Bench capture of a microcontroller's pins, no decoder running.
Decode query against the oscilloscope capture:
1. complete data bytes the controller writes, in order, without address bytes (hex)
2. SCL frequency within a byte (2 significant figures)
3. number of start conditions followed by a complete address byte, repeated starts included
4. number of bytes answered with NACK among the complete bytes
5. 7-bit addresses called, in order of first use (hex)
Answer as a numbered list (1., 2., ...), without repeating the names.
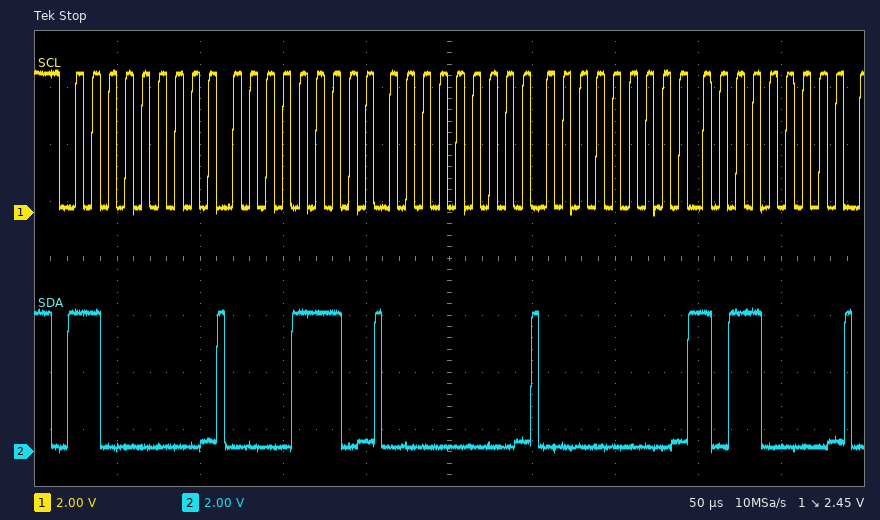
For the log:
1. 0E 00 00 B0
2. 100 kHz
3. 1
4. 0
5. 0x60
